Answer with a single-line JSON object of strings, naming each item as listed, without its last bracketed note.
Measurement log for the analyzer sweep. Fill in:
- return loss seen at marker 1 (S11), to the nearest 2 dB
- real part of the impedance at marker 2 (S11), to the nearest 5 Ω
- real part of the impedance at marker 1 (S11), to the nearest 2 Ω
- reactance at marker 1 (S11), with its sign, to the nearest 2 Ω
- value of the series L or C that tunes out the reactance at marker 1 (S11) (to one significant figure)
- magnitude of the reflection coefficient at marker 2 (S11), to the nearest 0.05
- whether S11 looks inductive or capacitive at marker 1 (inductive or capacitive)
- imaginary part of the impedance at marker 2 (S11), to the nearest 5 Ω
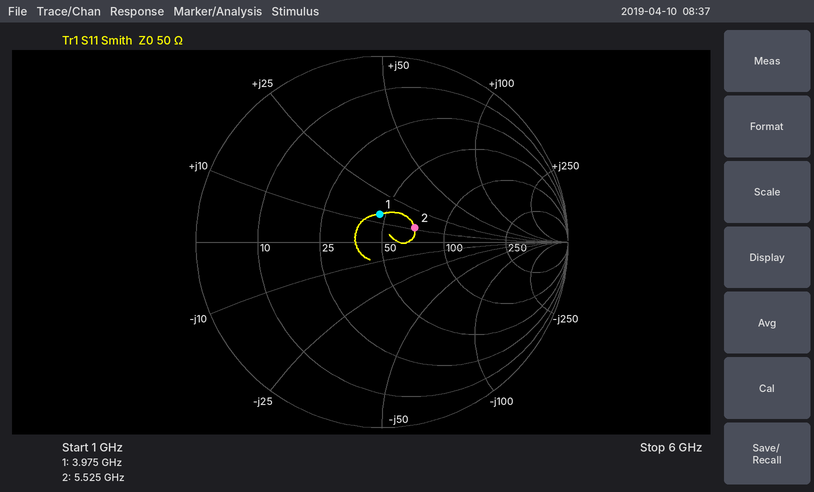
{"return loss seen at marker 1 (S11), to the nearest 2 dB": "16 dB", "real part of the impedance at marker 2 (S11), to the nearest 5 Ω": "70 Ω", "real part of the impedance at marker 1 (S11), to the nearest 2 Ω": "46 Ω", "reactance at marker 1 (S11), with its sign, to the nearest 2 Ω": "+14 Ω", "value of the series L or C that tunes out the reactance at marker 1 (S11)": "3 pF", "magnitude of the reflection coefficient at marker 2 (S11), to the nearest 0.05": "0.20", "whether S11 looks inductive or capacitive at marker 1": "inductive", "imaginary part of the impedance at marker 2 (S11), to the nearest 5 Ω": "+10 Ω"}
